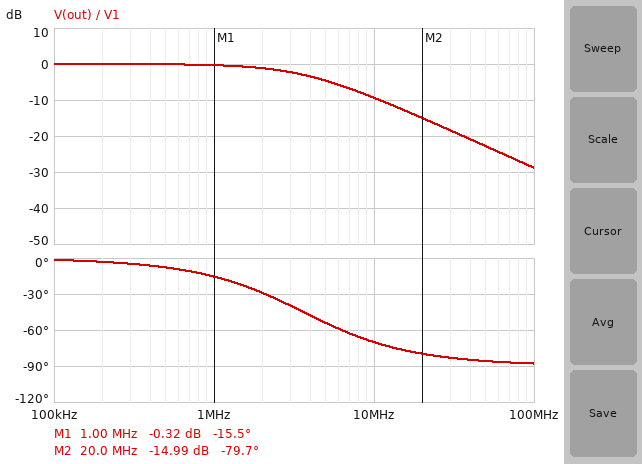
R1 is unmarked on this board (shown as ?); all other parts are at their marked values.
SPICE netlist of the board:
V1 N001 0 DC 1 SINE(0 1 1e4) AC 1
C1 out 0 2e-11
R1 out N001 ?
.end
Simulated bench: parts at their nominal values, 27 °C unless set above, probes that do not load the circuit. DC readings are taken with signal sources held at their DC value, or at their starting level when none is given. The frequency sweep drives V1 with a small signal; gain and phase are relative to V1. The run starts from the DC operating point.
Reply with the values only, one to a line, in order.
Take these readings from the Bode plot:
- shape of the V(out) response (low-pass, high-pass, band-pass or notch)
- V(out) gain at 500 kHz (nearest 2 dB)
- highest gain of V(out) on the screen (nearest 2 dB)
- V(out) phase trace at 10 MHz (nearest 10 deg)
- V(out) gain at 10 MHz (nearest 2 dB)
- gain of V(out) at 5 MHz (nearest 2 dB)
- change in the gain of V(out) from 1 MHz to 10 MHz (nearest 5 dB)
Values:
low-pass
0 dB
0 dB
-70 deg
-10 dB
-4 dB
-10 dB
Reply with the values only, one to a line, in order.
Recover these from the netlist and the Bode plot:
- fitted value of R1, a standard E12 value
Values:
2.2 kΩ
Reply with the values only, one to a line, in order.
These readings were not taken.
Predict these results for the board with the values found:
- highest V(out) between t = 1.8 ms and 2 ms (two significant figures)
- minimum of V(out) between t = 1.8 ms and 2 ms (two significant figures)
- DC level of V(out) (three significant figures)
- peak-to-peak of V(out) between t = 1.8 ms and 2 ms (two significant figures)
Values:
1.0 V
-1.0 V
1.00 V
2.0 V
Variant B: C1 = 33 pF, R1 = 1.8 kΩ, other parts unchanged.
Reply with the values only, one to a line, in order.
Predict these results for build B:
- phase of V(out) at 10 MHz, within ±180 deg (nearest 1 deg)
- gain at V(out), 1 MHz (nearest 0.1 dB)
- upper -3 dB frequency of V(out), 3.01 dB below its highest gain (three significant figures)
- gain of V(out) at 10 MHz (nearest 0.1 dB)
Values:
-75 deg
-0.6 dB
2.68 MHz
-11.7 dB
